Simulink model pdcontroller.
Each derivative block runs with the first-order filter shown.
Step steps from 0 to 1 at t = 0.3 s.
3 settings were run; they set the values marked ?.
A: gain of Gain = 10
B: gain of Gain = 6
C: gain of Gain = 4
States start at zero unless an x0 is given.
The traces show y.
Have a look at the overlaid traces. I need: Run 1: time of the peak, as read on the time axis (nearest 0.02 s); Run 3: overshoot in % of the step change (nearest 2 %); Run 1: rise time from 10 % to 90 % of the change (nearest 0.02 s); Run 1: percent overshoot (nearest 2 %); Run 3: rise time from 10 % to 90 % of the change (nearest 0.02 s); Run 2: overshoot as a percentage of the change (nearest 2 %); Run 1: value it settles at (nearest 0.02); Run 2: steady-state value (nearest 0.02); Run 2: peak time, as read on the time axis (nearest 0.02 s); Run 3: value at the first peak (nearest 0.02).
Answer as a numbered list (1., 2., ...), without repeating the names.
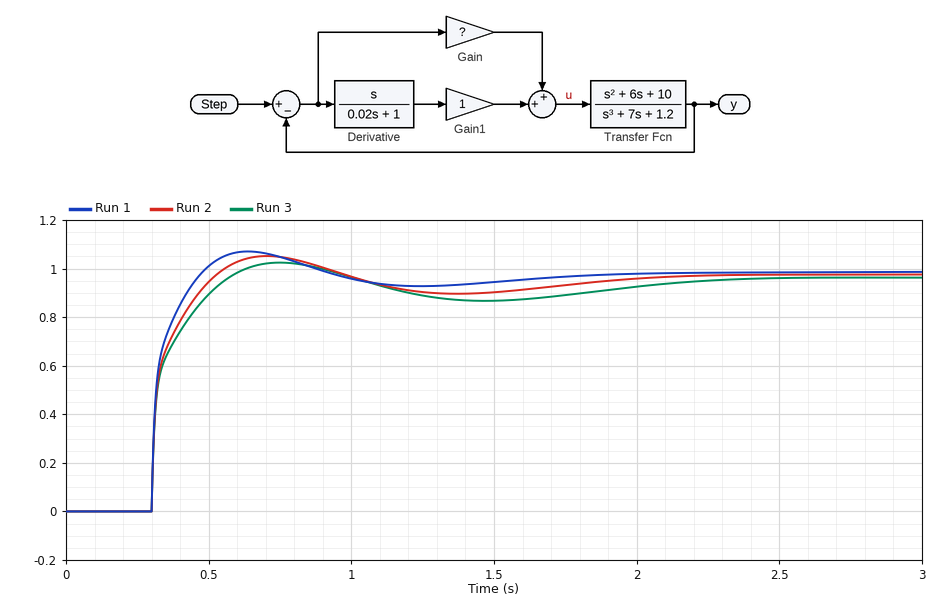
1. 0.64 s
2. 6 %
3. 0.12 s
4. 8 %
5. 0.18 s
6. 8 %
7. 0.98
8. 0.98
9. 0.70 s
10. 1.02
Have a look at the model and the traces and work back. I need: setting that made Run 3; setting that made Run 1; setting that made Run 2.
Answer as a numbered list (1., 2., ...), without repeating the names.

1. C
2. A
3. B
